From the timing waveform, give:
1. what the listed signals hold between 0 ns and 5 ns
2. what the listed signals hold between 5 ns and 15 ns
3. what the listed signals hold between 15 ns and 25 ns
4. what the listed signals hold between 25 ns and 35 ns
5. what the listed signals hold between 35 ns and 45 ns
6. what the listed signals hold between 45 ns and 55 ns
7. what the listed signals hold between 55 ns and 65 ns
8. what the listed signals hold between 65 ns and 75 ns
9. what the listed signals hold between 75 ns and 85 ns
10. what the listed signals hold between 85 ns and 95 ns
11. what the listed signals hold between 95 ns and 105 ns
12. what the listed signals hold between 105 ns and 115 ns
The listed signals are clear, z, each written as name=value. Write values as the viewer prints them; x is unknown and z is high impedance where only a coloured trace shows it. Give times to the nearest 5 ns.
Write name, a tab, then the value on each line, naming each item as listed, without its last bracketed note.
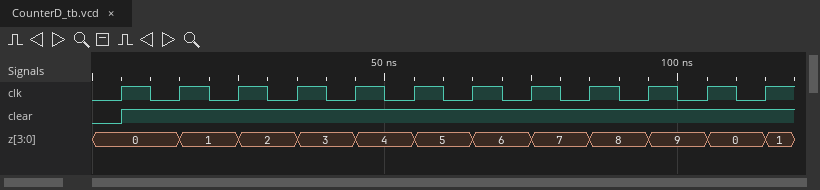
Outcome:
what the listed signals hold between 0 ns and 5 ns	clear=0, z=0
what the listed signals hold between 5 ns and 15 ns	clear=1, z=0
what the listed signals hold between 15 ns and 25 ns	clear=1, z=1
what the listed signals hold between 25 ns and 35 ns	clear=1, z=2
what the listed signals hold between 35 ns and 45 ns	clear=1, z=3
what the listed signals hold between 45 ns and 55 ns	clear=1, z=4
what the listed signals hold between 55 ns and 65 ns	clear=1, z=5
what the listed signals hold between 65 ns and 75 ns	clear=1, z=6
what the listed signals hold between 75 ns and 85 ns	clear=1, z=7
what the listed signals hold between 85 ns and 95 ns	clear=1, z=8
what the listed signals hold between 95 ns and 105 ns	clear=1, z=9
what the listed signals hold between 105 ns and 115 ns	clear=1, z=0
